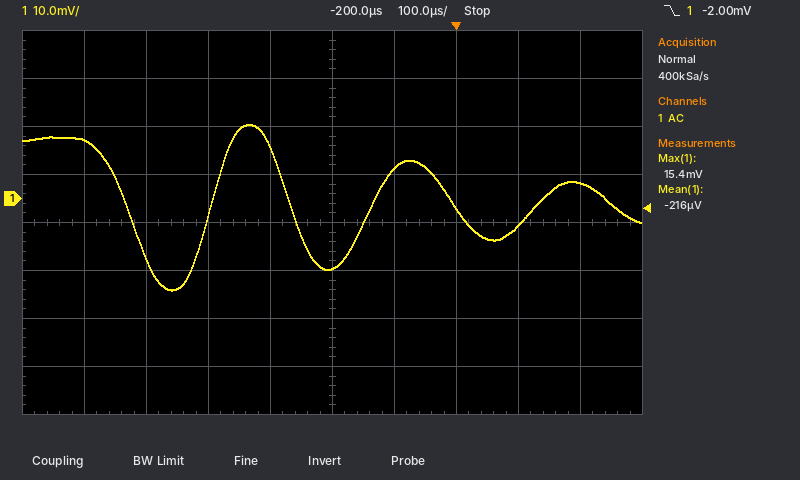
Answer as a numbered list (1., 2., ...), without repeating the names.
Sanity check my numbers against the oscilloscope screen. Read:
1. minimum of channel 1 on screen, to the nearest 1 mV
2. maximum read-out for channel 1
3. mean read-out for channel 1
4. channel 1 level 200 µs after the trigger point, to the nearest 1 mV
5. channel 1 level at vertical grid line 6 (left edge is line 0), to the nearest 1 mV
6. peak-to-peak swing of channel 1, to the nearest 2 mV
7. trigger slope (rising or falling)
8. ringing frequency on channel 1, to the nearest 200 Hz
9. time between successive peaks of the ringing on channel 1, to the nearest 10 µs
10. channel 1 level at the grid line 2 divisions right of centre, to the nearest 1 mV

1. -19 mV
2. 15.4 mV
3. -216 µV
4. 3 mV
5. 6 mV
6. 34 mV
7. falling
8. 3.8 kHz
9. 260 µs
10. -2 mV
